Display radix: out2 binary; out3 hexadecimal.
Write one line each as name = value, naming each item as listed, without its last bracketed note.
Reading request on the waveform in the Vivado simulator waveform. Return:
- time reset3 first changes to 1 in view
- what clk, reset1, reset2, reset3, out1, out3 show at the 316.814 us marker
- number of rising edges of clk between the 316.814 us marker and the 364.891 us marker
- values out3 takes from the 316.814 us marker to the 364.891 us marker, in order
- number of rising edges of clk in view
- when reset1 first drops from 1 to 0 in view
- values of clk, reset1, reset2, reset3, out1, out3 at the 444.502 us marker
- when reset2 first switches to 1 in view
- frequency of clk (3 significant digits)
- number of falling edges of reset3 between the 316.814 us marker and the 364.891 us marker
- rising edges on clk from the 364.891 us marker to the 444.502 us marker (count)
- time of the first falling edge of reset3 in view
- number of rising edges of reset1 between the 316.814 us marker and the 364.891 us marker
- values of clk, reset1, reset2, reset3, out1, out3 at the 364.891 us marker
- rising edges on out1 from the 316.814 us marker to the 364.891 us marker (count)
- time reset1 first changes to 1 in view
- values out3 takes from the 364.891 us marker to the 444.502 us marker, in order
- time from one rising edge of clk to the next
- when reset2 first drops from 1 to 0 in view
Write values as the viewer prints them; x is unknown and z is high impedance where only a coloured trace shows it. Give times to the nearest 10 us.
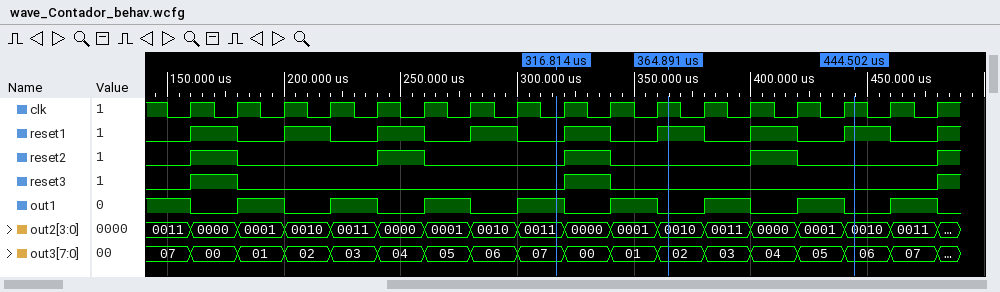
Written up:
time reset3 first changes to 1 in view = 160 us
what clk, reset1, reset2, reset3, out1, out3 show at the 316.814 us marker = clk=0, reset1=0, reset2=0, reset3=0, out1=1, out3=07
number of rising edges of clk between the 316.814 us marker and the 364.891 us marker = 3
values out3 takes from the 316.814 us marker to the 364.891 us marker, in order = 07, 00, 01, 02
number of rising edges of clk in view = 17
when reset1 first drops from 1 to 0 in view = 180 us
values of clk, reset1, reset2, reset3, out1, out3 at the 444.502 us marker = clk=1, reset1=1, reset2=0, reset3=0, out1=0, out3=06
when reset2 first switches to 1 in view = 160 us
frequency of clk = 50.0 kHz
number of falling edges of reset3 between the 316.814 us marker and the 364.891 us marker = 1
rising edges on clk from the 364.891 us marker to the 444.502 us marker = 4
time of the first falling edge of reset3 in view = 180 us
number of rising edges of reset1 between the 316.814 us marker and the 364.891 us marker = 2
values of clk, reset1, reset2, reset3, out1, out3 at the 364.891 us marker = clk=1, reset1=1, reset2=0, reset3=0, out1=0, out3=02
rising edges on out1 from the 316.814 us marker to the 364.891 us marker = 1
time reset1 first changes to 1 in view = 160 us
values out3 takes from the 364.891 us marker to the 444.502 us marker, in order = 02, 03, 04, 05, 06
time from one rising edge of clk to the next = 20 us
when reset2 first drops from 1 to 0 in view = 180 us
